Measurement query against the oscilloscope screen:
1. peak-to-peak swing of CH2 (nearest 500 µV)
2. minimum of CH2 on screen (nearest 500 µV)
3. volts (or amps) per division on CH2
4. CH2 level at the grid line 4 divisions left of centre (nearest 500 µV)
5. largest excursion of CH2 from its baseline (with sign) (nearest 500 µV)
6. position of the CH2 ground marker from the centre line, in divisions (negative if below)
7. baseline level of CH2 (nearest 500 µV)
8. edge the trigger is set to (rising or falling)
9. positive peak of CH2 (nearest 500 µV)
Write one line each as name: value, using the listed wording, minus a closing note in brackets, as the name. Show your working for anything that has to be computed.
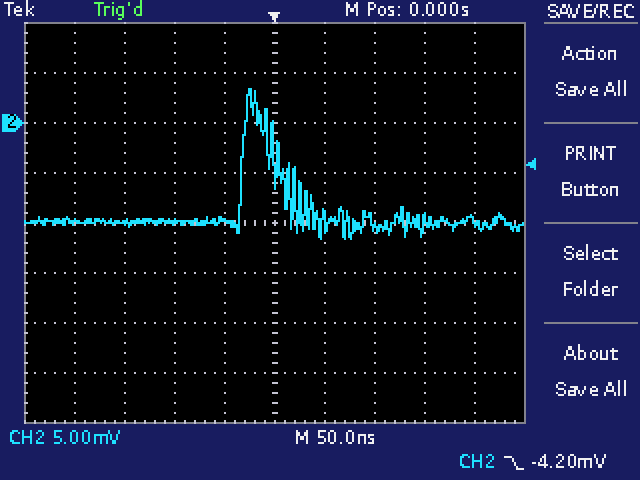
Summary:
peak-to-peak swing of CH2: 3.5 mV − (-11.5 mV) = 15.0 mV
minimum of CH2 on screen: -11.5 mV
volts (or amps) per division on CH2: 5 mV
CH2 level at the grid line 4 divisions left of centre: -10.0 mV
largest excursion of CH2 from its baseline (with sign): 3.5 mV − (-10.0 mV) = +13.5 mV
position of the CH2 ground marker from the centre line, in divisions: +2.0 div
baseline level of CH2: -10.0 mV
edge the trigger is set to: falling
positive peak of CH2: 3.5 mV
